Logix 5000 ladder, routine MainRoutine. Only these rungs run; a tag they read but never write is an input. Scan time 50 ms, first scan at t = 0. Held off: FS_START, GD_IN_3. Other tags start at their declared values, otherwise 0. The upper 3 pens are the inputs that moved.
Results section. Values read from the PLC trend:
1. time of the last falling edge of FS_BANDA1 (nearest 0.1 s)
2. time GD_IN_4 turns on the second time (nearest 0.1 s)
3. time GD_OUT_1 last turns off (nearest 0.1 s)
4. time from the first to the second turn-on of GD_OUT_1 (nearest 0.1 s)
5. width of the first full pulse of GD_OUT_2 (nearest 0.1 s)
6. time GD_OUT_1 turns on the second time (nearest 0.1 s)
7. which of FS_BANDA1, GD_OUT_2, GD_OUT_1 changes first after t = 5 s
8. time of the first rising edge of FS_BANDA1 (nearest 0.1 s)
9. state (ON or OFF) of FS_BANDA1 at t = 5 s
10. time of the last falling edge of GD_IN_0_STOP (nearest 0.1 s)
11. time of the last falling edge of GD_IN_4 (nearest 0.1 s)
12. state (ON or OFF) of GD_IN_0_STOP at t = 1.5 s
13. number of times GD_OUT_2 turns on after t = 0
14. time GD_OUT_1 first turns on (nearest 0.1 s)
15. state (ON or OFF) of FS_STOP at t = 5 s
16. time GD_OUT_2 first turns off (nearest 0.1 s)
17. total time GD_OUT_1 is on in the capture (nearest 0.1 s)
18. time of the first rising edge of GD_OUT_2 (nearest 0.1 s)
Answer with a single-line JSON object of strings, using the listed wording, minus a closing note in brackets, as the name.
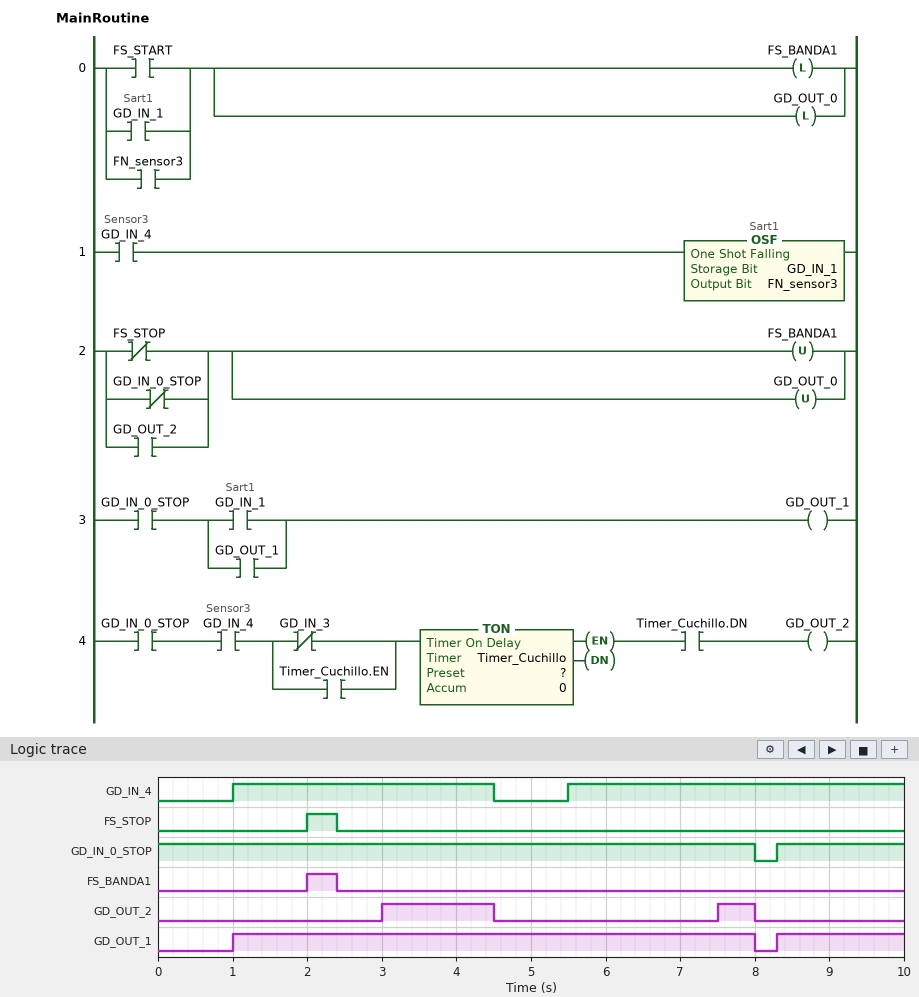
{"time of the last falling edge of FS_BANDA1": "2.4 s", "time GD_IN_4 turns on the second time": "5.5 s", "time GD_OUT_1 last turns off": "8.0 s", "time from the first to the second turn-on of GD_OUT_1": "7.3 s", "width of the first full pulse of GD_OUT_2": "1.5 s", "time GD_OUT_1 turns on the second time": "8.3 s", "which of FS_BANDA1, GD_OUT_2, GD_OUT_1 changes first after t = 5 s": "GD_OUT_2", "time of the first rising edge of FS_BANDA1": "2.0 s", "state (ON or OFF) of FS_BANDA1 at t = 5 s": "OFF", "time of the last falling edge of GD_IN_0_STOP": "8.0 s", "time of the last falling edge of GD_IN_4": "4.5 s", "state (ON or OFF) of GD_IN_0_STOP at t = 1.5 s": "ON", "number of times GD_OUT_2 turns on after t = 0": "2", "time GD_OUT_1 first turns on": "1.0 s", "state (ON or OFF) of FS_STOP at t = 5 s": "OFF", "time GD_OUT_2 first turns off": "4.5 s", "total time GD_OUT_1 is on in the capture": "8.7 s", "time of the first rising edge of GD_OUT_2": "3.0 s"}
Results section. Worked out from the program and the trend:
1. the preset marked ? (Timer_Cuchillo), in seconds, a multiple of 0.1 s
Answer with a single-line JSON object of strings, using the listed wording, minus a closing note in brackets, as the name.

{"the preset marked ? (Timer_Cuchillo), in seconds, a multiple of 0.1 s": "2.0 s"}
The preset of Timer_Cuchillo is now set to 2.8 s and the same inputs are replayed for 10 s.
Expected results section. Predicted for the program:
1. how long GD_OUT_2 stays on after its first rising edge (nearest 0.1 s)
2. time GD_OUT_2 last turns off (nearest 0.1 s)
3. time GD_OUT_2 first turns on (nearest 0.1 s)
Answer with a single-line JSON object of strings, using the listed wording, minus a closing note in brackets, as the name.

{"how long GD_OUT_2 stays on after its first rising edge": "0.7 s", "time GD_OUT_2 last turns off": "4.5 s", "time GD_OUT_2 first turns on": "3.8 s"}
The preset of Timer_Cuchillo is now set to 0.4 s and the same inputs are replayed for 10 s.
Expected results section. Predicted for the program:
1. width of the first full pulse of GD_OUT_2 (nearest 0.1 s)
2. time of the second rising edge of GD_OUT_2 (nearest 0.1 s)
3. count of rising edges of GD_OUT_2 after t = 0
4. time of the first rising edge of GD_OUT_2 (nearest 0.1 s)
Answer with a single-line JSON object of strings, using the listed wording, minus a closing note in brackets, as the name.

{"width of the first full pulse of GD_OUT_2": "3.1 s", "time of the second rising edge of GD_OUT_2": "5.9 s", "count of rising edges of GD_OUT_2 after t = 0": "3", "time of the first rising edge of GD_OUT_2": "1.4 s"}
